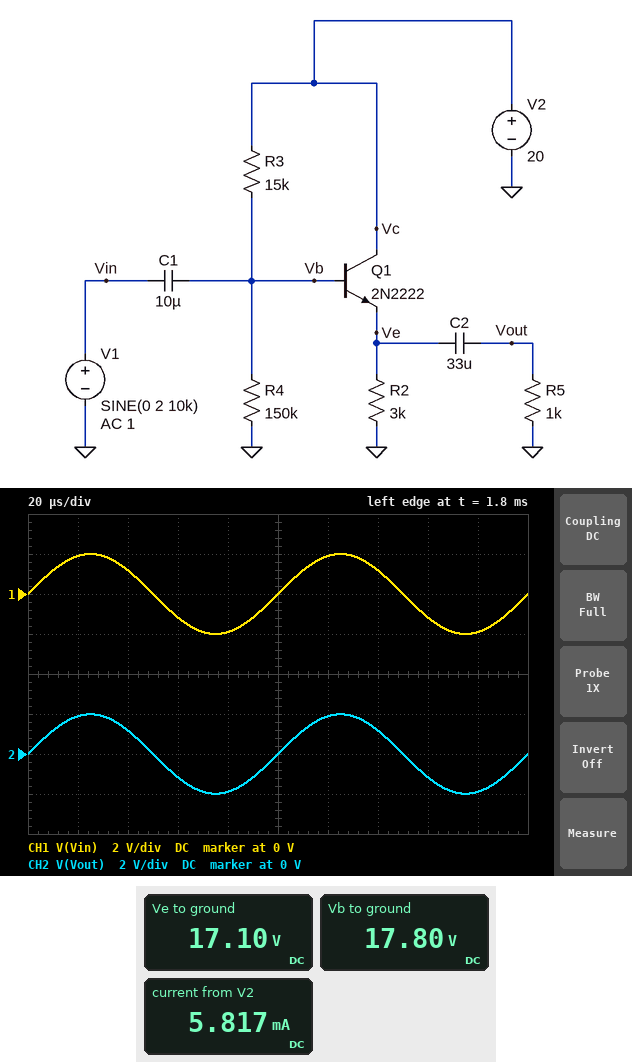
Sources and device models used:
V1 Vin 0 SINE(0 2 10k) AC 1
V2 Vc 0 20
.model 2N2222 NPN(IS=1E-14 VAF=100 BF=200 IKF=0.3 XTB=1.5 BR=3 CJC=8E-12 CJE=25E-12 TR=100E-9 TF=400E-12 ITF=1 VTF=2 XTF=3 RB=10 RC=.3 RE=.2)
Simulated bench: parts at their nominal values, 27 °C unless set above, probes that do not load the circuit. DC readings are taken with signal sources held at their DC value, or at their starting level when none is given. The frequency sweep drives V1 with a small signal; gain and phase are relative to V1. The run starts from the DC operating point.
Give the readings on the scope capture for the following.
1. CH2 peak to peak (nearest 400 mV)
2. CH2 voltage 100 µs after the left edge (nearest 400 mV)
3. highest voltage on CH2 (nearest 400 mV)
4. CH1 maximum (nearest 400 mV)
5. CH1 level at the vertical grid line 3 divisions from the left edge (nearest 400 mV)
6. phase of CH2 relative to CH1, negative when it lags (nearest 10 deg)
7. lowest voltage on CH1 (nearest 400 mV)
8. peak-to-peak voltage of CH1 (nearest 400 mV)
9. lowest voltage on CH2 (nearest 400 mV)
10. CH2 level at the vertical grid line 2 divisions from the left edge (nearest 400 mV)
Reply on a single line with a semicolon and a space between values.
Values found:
4.0 V; 0 V; 2.0 V; 2.0 V; -1.2 V; 0 deg; -2.0 V; 4.0 V; -2.0 V; 1.2 V
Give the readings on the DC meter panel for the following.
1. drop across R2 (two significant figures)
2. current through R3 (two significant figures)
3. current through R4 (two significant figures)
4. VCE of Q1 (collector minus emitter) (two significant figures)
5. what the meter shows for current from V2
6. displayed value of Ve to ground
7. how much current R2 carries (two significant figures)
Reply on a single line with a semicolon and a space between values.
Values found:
17 V; 150 µA; 120 µA; 2.9 V; 5.817 mA; 17.10 V; 5.7 mA
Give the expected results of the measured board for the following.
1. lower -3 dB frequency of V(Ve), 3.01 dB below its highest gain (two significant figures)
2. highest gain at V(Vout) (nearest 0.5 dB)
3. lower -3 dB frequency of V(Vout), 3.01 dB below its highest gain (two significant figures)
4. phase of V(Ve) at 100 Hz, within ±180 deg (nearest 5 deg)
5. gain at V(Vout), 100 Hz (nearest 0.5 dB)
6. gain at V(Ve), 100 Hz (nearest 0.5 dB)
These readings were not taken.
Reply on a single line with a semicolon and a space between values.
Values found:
1.2 Hz; 0 dB; 5.2 Hz; 0 deg; 0 dB; 0 dB
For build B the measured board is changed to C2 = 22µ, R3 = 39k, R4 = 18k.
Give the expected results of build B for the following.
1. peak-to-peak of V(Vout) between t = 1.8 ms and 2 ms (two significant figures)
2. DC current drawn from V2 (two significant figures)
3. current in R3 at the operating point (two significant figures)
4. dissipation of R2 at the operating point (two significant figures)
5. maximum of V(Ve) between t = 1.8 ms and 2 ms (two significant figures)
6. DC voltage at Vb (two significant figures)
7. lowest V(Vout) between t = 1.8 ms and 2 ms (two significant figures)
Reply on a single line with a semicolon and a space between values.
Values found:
3.4 V; 2.2 mA; 350 µA; 10 mW; 7.5 V; 6.2 V; -1.4 V
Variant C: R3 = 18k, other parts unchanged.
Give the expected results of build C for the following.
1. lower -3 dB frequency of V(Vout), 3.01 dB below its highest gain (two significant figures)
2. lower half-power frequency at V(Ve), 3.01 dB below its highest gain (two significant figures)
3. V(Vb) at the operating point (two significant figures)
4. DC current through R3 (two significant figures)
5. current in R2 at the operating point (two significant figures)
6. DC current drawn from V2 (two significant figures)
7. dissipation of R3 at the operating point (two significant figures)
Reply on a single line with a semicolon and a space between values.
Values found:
5.1 Hz; 1.0 Hz; 17 V; 140 µA; 5.6 mA; 5.7 mA; 370 µW
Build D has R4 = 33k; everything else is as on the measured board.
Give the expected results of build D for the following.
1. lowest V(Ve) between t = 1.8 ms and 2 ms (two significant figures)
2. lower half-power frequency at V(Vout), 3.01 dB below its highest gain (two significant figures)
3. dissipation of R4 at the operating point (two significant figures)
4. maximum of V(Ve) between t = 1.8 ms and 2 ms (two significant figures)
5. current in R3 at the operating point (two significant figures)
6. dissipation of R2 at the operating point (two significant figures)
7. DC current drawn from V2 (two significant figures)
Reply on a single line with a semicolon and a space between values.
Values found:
11 V; 5.3 Hz; 5.6 mW; 15 V; 430 µA; 55 mW; 4.7 mA
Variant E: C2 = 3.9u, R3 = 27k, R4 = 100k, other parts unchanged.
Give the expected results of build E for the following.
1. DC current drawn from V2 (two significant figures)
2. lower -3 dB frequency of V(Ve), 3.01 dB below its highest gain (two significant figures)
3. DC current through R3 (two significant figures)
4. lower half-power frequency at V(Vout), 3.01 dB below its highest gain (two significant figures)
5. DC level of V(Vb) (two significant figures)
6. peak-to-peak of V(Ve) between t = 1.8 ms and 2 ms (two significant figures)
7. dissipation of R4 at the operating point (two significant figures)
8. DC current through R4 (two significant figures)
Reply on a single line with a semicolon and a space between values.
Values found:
5.0 mA; 770 mHz; 180 µA; 41 Hz; 15 V; 4.0 V; 2.3 mW; 150 µA
